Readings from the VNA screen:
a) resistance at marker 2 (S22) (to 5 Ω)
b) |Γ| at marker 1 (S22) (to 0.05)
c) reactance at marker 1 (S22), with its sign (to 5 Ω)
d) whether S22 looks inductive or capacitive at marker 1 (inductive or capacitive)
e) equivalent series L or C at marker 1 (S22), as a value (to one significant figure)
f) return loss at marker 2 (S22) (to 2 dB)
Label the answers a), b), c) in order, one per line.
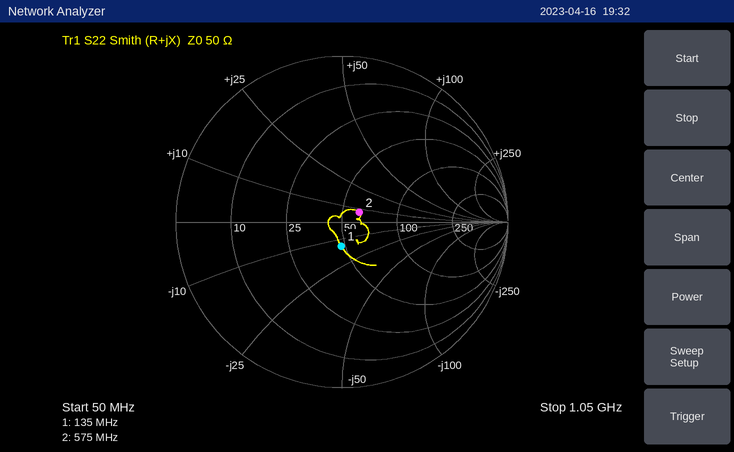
a) 60 Ω
b) 0.15
c) -15 Ω
d) capacitive
e) 80 pF
f) 18 dB
